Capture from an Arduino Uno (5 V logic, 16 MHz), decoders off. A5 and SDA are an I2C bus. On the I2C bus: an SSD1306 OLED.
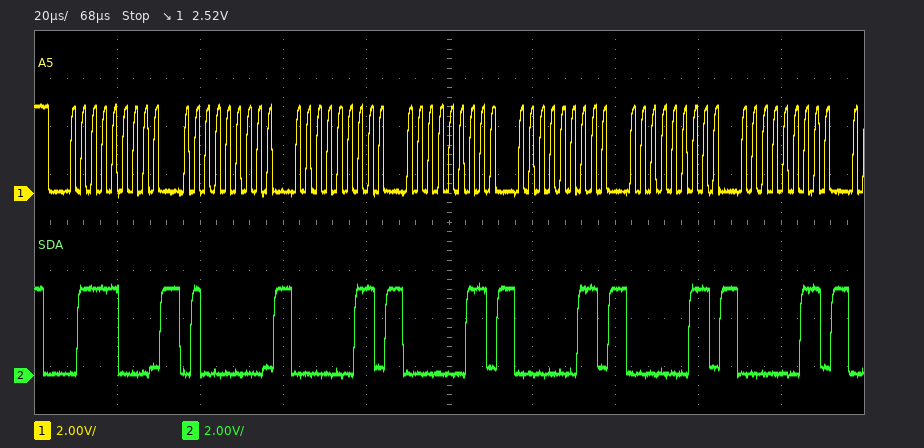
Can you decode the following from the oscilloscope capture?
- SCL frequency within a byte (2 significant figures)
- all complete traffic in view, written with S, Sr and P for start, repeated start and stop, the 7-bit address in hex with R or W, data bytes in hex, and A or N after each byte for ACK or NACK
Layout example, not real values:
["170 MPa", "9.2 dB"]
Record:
["400 kHz", "S 3CW A 40 A 03 A 03 A 03 A 03 A 03 A"]
